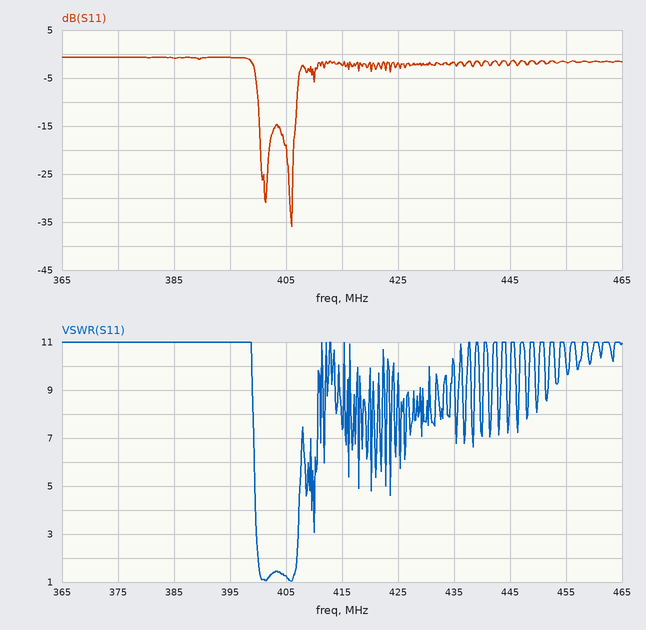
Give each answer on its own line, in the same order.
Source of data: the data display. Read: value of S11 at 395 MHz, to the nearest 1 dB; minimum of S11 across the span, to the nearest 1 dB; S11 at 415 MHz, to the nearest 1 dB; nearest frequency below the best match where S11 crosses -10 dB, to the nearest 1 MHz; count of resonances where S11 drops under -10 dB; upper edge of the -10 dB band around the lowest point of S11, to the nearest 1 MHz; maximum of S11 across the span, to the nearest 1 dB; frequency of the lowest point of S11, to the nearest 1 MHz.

-1 dB
-36 dB
-2 dB
400 MHz
2
407 MHz
-1 dB
406 MHz
